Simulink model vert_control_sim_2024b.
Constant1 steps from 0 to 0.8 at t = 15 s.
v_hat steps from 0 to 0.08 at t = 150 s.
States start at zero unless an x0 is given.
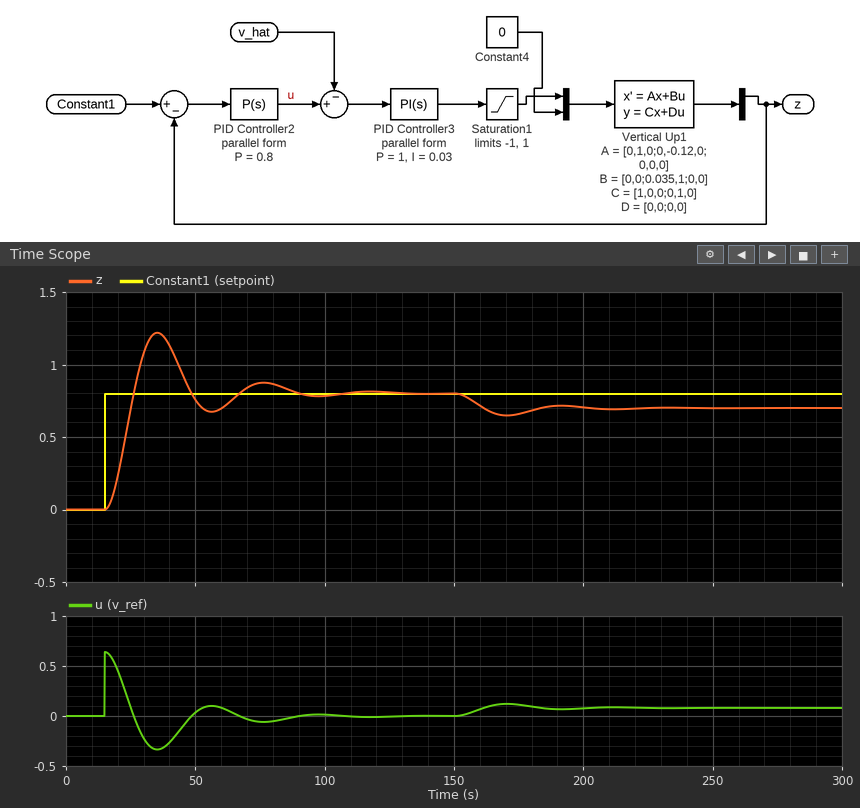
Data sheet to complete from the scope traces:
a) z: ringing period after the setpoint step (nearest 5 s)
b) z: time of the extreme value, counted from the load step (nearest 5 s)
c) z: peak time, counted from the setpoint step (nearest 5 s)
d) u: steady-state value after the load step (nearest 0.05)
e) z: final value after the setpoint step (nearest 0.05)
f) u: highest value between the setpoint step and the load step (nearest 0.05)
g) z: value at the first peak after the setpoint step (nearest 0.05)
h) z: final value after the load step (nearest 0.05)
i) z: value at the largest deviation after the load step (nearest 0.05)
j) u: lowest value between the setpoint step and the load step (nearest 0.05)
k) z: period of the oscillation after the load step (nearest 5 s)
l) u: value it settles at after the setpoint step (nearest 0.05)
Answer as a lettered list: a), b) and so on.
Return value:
a) 40 s
b) 20 s
c) 20 s
d) 0.10
e) 0.80
f) 0.65
g) 1.20
h) 0.70
i) 0.65
j) -0.35
k) 40 s
l) 0.00
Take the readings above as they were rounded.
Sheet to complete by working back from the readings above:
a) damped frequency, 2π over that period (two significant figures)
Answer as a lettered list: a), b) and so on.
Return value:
a) 0.16 rad/s
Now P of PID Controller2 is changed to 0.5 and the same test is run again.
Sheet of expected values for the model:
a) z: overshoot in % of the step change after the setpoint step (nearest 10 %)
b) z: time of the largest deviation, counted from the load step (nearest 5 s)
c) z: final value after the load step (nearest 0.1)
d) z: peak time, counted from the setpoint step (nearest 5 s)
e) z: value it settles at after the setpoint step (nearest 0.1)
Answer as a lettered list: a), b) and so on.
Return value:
a) 50 %
b) 25 s
c) 0.6
d) 25 s
e) 0.8
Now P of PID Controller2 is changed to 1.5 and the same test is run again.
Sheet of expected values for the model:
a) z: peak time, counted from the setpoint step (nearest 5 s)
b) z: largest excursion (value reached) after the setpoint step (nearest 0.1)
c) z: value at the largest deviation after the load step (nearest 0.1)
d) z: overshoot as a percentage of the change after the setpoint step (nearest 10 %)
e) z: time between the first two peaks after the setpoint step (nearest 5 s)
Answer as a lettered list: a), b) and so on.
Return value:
a) 15 s
b) 1.3
c) 0.7
d) 60 %
e) 30 s
